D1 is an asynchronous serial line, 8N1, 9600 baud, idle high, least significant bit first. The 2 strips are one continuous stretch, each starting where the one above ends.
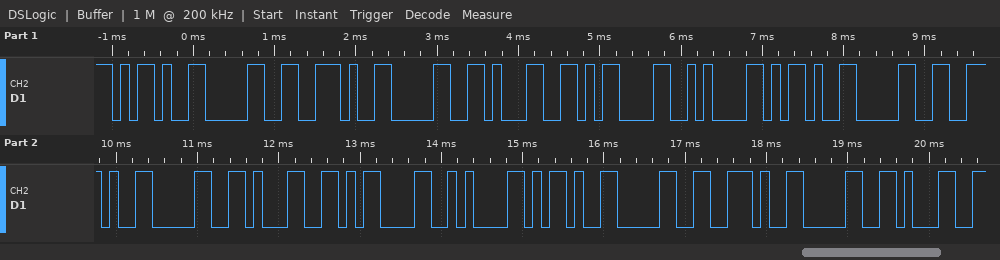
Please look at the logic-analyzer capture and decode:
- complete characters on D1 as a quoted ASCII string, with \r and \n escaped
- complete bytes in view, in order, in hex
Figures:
"-0.01\r\n-0.01\r\n-0.01"
2D 30 2E 30 31 0D 0A 2D 30 2E 30 31 0D 0A 2D 30 2E 30 31
